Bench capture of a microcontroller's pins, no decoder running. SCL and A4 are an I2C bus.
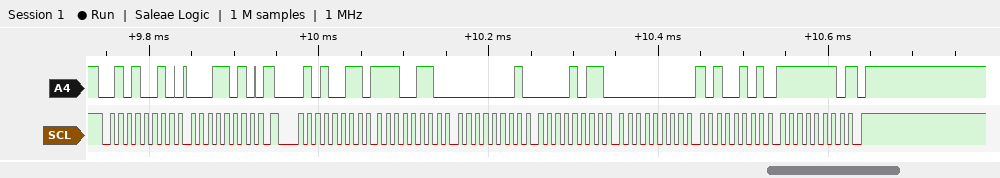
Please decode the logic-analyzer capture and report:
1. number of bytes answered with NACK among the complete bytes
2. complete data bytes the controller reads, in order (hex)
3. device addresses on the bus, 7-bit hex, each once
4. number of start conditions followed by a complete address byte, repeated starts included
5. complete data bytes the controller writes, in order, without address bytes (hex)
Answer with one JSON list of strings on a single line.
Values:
["1", "E6 01 0B 00 A5 FE", "0x29", "2", "1A"]
